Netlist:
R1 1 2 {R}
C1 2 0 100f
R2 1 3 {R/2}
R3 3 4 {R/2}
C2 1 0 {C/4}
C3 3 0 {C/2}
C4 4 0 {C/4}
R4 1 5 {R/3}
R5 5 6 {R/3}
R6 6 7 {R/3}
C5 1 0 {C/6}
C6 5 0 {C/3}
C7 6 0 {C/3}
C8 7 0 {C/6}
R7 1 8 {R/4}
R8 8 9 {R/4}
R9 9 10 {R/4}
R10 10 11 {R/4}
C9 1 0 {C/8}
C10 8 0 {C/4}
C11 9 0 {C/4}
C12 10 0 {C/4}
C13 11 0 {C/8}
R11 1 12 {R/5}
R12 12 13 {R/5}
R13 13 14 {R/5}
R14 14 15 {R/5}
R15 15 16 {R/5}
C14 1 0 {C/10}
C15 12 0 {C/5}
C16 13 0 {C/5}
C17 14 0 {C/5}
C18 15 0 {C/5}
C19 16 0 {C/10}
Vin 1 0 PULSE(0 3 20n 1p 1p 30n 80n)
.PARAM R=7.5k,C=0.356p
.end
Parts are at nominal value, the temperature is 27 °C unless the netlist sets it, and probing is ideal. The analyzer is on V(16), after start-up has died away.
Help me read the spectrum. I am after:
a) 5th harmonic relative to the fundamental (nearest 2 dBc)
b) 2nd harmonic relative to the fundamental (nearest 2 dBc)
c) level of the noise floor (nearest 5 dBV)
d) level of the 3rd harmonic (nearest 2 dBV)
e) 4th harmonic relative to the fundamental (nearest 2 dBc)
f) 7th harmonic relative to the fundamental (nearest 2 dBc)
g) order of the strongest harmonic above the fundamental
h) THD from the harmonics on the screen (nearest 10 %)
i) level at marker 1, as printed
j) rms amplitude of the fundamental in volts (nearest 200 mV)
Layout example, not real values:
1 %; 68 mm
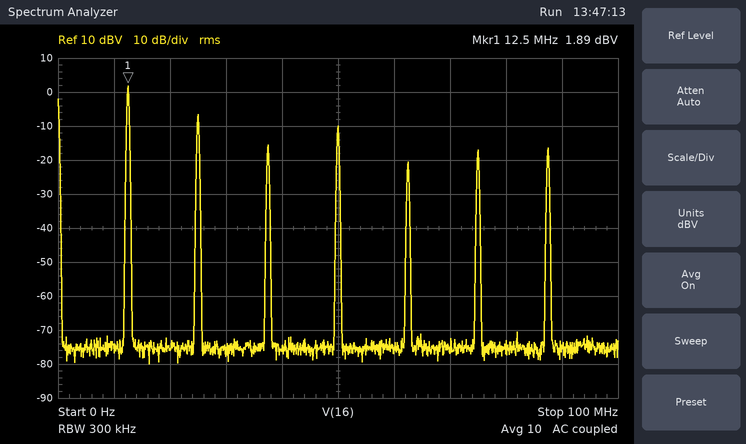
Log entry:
-22 dBc; -8 dBc; -75 dBV; -16 dBV; -12 dBc; -18 dBc; 2; 50 %; 1.89 dBV; 1.2 V
